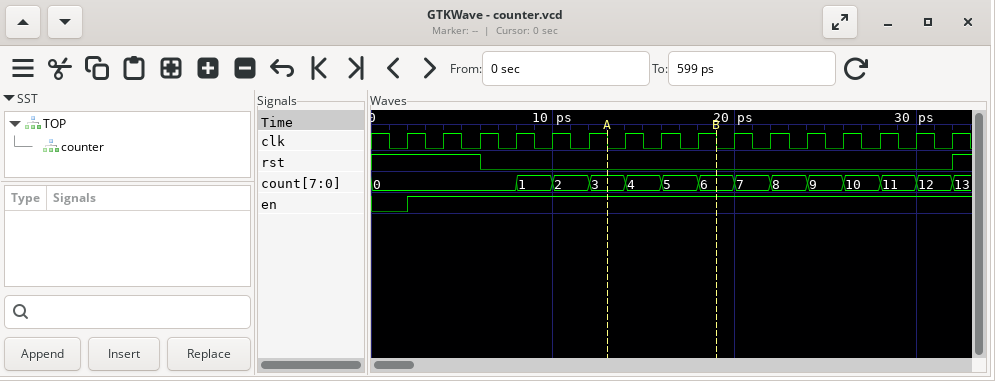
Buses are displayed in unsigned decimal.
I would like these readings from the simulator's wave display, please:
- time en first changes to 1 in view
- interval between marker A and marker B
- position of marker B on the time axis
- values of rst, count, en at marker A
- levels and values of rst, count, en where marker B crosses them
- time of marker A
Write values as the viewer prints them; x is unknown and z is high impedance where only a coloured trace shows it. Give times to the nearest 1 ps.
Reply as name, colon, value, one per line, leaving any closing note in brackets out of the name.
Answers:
time en first changes to 1 in view: 2 ps
interval between marker A and marker B: 6 ps
position of marker B on the time axis: 19 ps
values of rst, count, en at marker A: rst=0, count=3, en=1
levels and values of rst, count, en where marker B crosses them: rst=0, count=6, en=1
time of marker A: 13 ps
